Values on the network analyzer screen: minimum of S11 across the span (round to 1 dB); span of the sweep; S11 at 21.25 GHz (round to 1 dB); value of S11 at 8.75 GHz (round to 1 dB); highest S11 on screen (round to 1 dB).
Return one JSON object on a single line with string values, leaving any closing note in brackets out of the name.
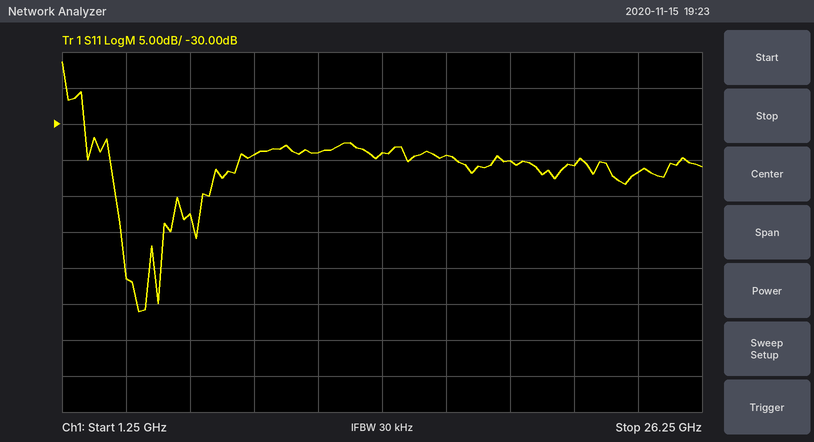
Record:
{"minimum of S11 across the span": "-56 dB", "span of the sweep": "25 GHz", "S11 at 21.25 GHz": "-36 dB", "value of S11 at 8.75 GHz": "-34 dB", "highest S11 on screen": "-21 dB"}
